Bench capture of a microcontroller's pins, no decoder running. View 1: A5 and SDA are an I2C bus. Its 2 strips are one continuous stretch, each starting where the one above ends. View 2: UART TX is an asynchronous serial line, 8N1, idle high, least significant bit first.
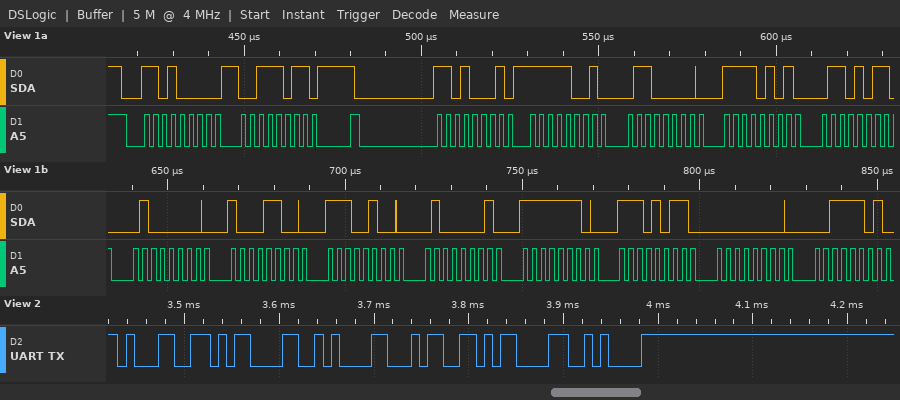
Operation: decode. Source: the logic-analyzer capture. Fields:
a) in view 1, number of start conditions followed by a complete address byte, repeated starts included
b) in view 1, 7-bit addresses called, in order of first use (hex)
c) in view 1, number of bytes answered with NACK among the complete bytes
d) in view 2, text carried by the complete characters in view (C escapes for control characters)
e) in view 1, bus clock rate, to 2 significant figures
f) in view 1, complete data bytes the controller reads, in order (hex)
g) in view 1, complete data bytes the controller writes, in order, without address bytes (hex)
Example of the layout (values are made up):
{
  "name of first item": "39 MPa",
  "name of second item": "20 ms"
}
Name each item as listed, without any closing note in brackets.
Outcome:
{
  "in view 1, number of start conditions followed by a complete address byte, repeated starts included": "2",
  "in view 1, 7-bit addresses called, in order of first use": "0x68",
  "in view 1, number of bytes answered with NACK among the complete bytes": "0",
  "in view 2, text carried by the complete characters in view": "\"1\\r\\n4\\r\\n\"",
  "in view 1, bus clock rate, to 2 significant figures": "400 kHz",
  "in view 1, complete data bytes the controller reads, in order": "F9 60 F5 6B 40 8C E4 41 FE EB 00 3D",
  "in view 1, complete data bytes the controller writes, in order, without address bytes": "3B"
}
